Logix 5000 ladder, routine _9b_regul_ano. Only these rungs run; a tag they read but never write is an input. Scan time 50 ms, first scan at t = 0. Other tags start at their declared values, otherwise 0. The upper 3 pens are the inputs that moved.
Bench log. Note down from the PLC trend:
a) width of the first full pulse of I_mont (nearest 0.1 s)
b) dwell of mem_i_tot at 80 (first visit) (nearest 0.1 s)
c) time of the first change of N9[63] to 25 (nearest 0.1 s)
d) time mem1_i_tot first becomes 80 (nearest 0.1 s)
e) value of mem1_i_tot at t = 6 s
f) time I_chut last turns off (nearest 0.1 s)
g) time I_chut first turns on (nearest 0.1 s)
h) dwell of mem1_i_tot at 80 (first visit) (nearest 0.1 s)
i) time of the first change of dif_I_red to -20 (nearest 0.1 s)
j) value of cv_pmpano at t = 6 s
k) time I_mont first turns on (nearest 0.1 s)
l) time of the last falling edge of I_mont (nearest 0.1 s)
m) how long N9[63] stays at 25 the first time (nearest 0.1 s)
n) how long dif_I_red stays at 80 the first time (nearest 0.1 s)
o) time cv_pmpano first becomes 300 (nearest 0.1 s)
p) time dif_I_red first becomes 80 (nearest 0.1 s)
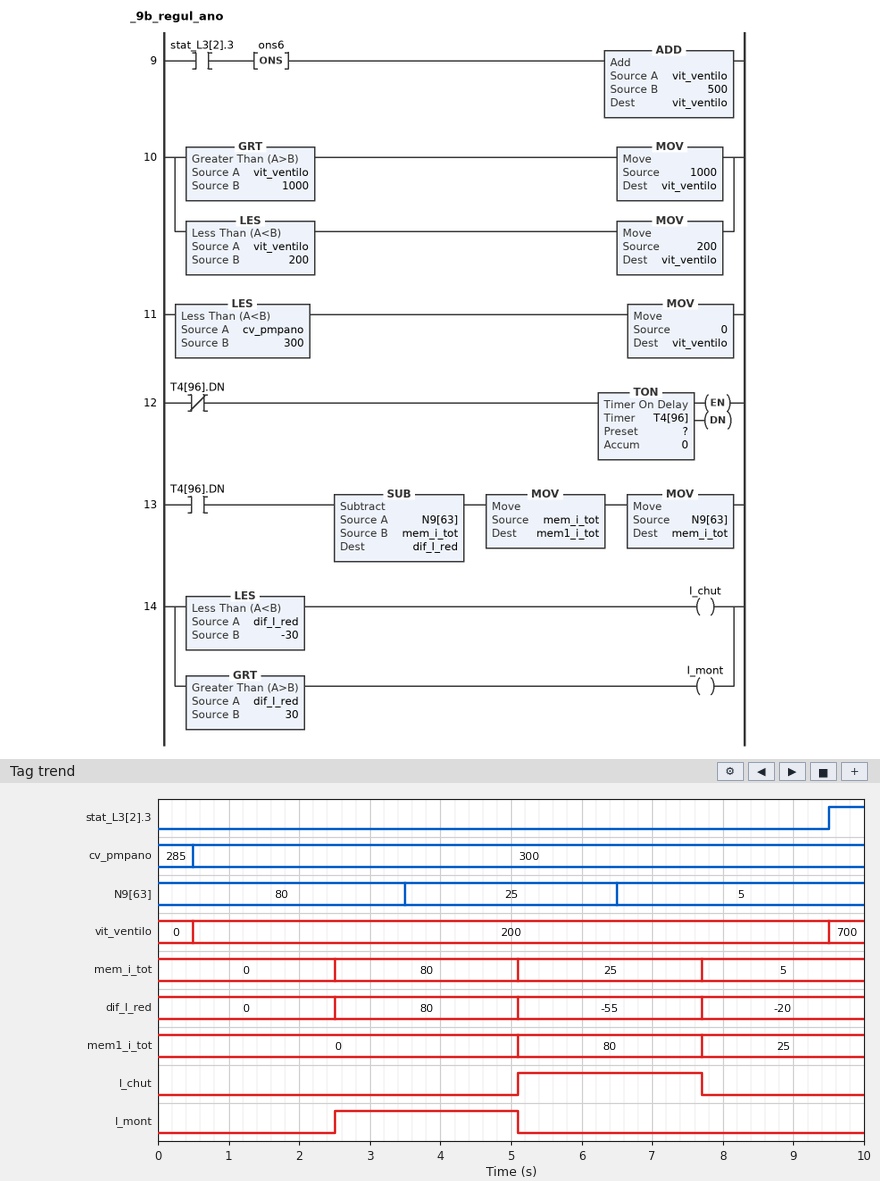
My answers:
2.6 s
2.6 s
3.5 s
5.1 s
80
7.7 s
5.1 s
2.6 s
7.7 s
300
2.5 s
5.1 s
3.0 s
2.6 s
0.5 s
2.5 s
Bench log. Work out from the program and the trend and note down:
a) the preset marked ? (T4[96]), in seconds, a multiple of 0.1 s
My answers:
2.5 s
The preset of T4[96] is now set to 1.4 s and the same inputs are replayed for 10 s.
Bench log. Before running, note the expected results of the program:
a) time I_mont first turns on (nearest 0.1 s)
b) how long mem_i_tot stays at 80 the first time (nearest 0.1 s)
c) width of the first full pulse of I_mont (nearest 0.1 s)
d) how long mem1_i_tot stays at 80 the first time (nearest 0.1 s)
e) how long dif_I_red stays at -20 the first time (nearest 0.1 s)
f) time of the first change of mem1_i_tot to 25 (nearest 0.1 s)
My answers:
1.4 s
3.0 s
1.5 s
3.0 s
1.5 s
5.9 s
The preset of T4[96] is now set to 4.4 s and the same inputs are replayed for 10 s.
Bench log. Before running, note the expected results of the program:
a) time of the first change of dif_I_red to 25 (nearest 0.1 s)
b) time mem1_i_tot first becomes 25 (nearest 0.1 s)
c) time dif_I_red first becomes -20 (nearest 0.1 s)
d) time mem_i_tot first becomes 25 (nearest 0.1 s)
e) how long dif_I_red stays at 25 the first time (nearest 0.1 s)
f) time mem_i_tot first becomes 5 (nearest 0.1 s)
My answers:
4.4 s
8.9 s
8.9 s
4.4 s
4.5 s
8.9 s
